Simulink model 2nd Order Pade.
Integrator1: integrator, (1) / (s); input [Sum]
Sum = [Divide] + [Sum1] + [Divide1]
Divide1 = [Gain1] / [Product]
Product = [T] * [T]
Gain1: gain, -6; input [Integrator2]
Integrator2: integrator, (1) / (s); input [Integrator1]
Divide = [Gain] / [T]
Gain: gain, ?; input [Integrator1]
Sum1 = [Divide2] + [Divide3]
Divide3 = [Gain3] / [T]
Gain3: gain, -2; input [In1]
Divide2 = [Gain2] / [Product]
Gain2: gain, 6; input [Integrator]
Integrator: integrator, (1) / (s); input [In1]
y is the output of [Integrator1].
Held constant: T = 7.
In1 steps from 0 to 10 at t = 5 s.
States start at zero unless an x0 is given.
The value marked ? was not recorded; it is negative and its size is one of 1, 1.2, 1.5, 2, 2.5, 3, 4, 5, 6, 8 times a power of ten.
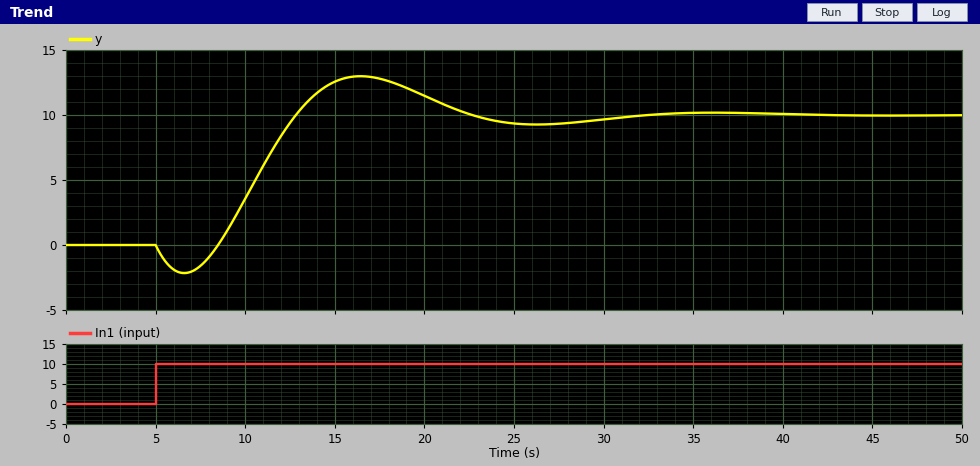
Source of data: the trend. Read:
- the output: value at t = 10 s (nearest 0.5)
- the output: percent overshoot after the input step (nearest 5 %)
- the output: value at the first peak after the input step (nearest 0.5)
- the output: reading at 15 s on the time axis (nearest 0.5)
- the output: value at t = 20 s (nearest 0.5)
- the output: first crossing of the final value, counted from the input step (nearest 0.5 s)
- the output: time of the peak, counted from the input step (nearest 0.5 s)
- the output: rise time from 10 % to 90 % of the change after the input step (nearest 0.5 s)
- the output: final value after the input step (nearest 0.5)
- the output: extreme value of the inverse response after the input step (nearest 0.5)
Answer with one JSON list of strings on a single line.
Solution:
["3.5", "30 %", "13.0", "12.5", "11.5", "8.0 s", "11.5 s", "3.5 s", "10.0", "-2.0"]
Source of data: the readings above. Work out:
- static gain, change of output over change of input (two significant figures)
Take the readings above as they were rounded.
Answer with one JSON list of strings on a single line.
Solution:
["1.0"]
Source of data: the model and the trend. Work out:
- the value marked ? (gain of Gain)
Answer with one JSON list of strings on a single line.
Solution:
["-2"]
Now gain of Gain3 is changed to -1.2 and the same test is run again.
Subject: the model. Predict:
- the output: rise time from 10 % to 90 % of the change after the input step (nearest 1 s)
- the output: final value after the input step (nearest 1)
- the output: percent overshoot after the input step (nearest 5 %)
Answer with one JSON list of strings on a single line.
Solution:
["4 s", "10", "25 %"]
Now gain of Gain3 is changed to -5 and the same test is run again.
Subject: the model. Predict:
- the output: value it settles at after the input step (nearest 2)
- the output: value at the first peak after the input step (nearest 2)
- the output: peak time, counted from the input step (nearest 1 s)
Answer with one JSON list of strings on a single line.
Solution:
["10", "14", "12 s"]
